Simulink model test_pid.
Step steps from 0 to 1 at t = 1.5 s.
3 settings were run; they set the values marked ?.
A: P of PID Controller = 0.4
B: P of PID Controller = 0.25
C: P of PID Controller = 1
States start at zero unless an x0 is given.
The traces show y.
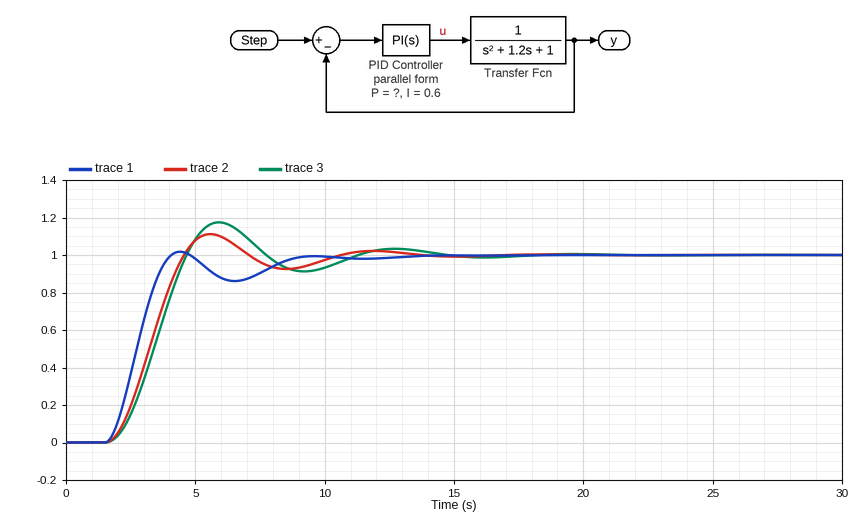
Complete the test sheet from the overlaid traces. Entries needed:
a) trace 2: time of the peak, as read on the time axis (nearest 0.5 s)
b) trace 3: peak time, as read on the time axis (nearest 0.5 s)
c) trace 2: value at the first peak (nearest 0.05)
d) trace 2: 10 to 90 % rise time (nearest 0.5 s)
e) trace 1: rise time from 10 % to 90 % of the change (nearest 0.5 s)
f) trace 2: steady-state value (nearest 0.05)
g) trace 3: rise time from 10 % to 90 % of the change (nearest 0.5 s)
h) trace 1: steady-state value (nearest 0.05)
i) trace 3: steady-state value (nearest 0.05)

5.5 s
6.0 s
1.10
2.0 s
1.5 s
1.00
2.0 s
1.00
1.00
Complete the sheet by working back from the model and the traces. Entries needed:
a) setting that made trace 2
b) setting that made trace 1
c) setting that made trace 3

A
C
B
